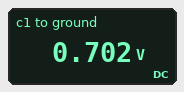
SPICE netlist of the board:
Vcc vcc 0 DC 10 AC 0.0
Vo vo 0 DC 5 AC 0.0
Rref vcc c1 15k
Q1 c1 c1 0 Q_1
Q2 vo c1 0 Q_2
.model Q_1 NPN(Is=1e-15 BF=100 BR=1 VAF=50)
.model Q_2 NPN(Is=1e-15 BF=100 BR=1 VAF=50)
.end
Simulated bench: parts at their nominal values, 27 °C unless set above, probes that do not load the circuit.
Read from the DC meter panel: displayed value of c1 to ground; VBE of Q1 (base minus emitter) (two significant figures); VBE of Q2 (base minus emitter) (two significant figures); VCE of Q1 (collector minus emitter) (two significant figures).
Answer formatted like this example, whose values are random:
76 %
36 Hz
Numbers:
0.702 V
700 mV
700 mV
700 mV
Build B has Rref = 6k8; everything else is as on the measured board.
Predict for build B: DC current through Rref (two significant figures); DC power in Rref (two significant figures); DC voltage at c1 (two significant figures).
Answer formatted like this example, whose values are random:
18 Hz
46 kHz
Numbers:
1.4 mA
13 mW
720 mV
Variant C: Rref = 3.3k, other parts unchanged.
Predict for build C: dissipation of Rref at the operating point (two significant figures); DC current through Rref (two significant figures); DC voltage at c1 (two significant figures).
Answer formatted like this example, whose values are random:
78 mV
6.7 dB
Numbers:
26 mW
2.8 mA
740 mV
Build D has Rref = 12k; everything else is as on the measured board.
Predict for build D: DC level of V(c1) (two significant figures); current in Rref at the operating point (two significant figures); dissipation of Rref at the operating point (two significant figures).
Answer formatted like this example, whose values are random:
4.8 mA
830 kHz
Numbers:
710 mV
770 µA
7.2 mW
